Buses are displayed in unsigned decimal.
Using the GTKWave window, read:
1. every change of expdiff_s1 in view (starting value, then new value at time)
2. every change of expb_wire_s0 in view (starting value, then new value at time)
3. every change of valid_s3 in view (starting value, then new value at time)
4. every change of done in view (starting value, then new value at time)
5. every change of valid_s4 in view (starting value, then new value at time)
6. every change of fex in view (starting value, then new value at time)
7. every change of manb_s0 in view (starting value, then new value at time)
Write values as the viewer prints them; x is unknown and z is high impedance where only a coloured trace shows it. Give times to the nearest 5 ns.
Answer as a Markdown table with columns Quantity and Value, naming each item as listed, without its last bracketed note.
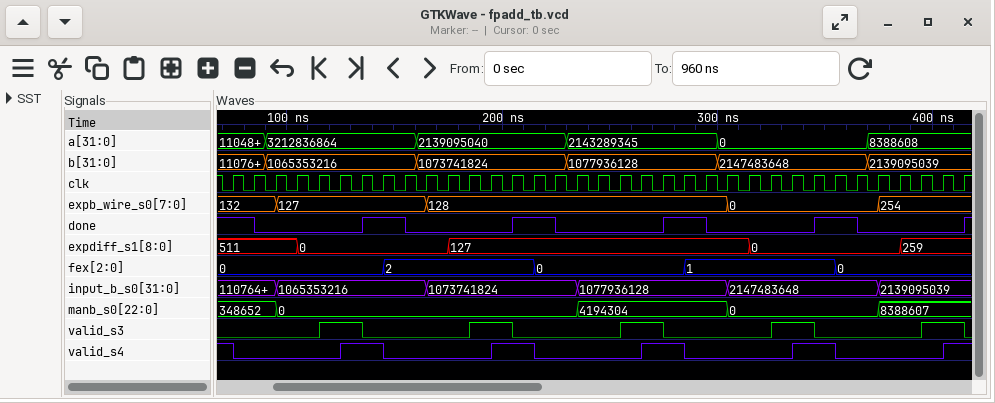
| Quantity | Value |
|---|---|
| every change of expdiff_s1 in view | 511, 0 at 105 ns, 127 at 175 ns, 0 at 315 ns, 259 at 385 ns |
| every change of expb_wire_s0 in view | 132, 127 at 95 ns, 128 at 165 ns, 0 at 305 ns, 254 at 375 ns |
| every change of valid_s3 in view | 0, 1 at 115 ns, 0 at 135 ns, 1 at 185 ns, 0 at 205 ns, 1 at 255 ns, 0 at 275 ns, 1 at 325 ns, 0 at 345 ns, 1 at 395 ns, 0 at 415 ns |
| every change of done in view | 1, 0 at 85 ns, 1 at 135 ns, 0 at 155 ns, 1 at 205 ns, 0 at 225 ns, 1 at 275 ns, 0 at 295 ns, 1 at 345 ns, 0 at 365 ns, 1 at 415 ns |
| every change of valid_s4 in view | 1, 0 at 75 ns, 1 at 125 ns, 0 at 145 ns, 1 at 195 ns, 0 at 215 ns, 1 at 265 ns, 0 at 285 ns, 1 at 335 ns, 0 at 355 ns, 1 at 405 ns |
| every change of fex in view | 0, 2 at 145 ns, 0 at 215 ns, 1 at 285 ns, 0 at 355 ns |
| every change of manb_s0 in view | 348652, 0 at 95 ns, 4194304 at 235 ns, 0 at 305 ns, 8388607 at 375 ns |
